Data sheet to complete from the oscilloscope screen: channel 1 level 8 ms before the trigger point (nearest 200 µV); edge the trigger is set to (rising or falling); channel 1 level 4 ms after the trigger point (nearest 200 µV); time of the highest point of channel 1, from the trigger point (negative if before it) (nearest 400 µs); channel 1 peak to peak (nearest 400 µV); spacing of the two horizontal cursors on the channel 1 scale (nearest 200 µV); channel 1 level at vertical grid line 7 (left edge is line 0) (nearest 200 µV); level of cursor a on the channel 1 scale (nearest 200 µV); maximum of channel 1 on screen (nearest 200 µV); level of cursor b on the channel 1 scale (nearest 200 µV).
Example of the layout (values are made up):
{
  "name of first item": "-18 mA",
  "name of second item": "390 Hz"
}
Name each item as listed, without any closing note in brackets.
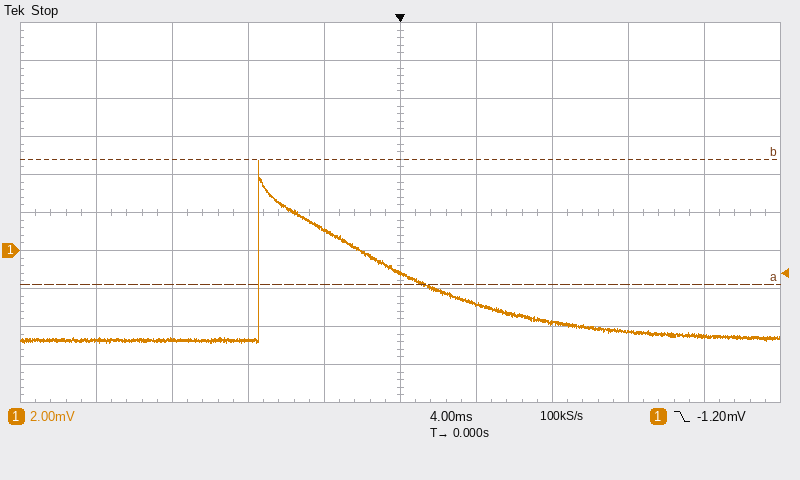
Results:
{
  "channel 1 level 8 ms before the trigger point": "-4.8 mV",
  "edge the trigger is set to": "falling",
  "channel 1 level 4 ms after the trigger point": "-2.8 mV",
  "time of the highest point of channel 1, from the trigger point (negative if before it)": "-7.6 ms",
  "channel 1 peak to peak": "9.6 mV",
  "spacing of the two horizontal cursors on the channel 1 scale": "6.6 mV",
  "channel 1 level at vertical grid line 7 (left edge is line 0)": "-3.8 mV",
  "level of cursor a on the channel 1 scale": "-1.8 mV",
  "maximum of channel 1 on screen": "4.8 mV",
  "level of cursor b on the channel 1 scale": "4.8 mV"
}
